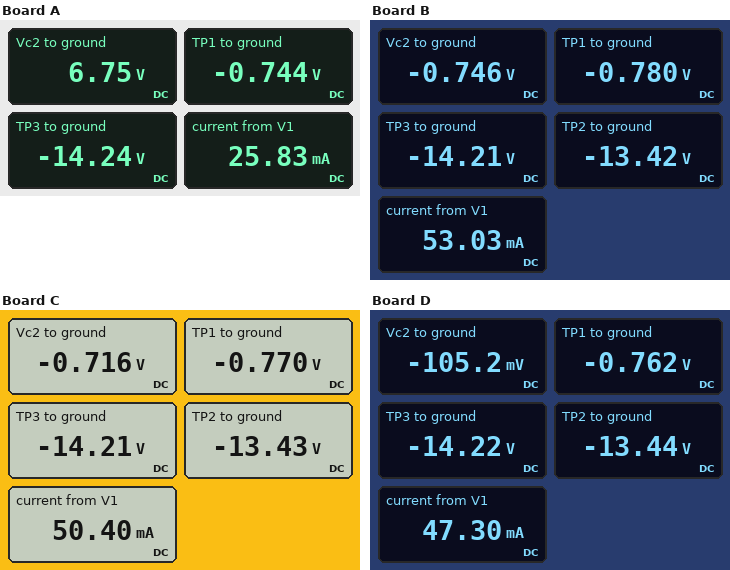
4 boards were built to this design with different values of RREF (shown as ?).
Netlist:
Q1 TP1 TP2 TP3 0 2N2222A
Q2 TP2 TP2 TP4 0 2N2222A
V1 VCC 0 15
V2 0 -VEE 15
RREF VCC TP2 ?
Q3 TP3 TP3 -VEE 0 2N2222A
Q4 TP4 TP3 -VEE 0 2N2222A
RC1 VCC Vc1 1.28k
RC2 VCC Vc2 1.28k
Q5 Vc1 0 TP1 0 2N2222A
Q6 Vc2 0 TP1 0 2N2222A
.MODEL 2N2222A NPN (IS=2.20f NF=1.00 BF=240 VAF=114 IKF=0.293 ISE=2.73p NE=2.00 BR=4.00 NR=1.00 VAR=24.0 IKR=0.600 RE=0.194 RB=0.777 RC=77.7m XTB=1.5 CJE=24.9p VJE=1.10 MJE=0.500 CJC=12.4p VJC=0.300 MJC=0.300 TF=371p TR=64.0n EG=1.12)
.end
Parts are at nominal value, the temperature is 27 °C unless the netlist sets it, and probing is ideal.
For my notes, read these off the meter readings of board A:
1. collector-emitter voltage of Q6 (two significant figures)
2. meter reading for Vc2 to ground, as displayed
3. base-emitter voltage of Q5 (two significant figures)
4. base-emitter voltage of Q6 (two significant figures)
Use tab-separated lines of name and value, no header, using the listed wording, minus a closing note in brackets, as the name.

collector-emitter voltage of Q6	7.5 V
meter reading for Vc2 to ground, as displayed	6.75 V
base-emitter voltage of Q5	740 mV
base-emitter voltage of Q6	740 mV
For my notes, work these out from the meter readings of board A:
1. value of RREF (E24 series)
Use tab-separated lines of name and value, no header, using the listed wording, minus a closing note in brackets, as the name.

value of RREF	2.2 kΩ
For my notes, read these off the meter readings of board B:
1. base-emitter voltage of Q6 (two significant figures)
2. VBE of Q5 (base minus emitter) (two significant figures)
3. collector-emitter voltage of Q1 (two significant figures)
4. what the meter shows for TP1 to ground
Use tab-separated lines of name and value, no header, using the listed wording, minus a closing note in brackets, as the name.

base-emitter voltage of Q6	780 mV
VBE of Q5 (base minus emitter)	780 mV
collector-emitter voltage of Q1	13 V
what the meter shows for TP1 to ground	-0.780 V
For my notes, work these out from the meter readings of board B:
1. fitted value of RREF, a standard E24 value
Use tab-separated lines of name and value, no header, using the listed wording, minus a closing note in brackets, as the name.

fitted value of RREF, a standard E24 value	1 kΩ
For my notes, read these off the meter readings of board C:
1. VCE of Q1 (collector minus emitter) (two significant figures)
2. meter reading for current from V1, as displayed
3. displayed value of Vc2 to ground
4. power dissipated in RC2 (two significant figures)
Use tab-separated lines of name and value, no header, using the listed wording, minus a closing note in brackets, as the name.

VCE of Q1 (collector minus emitter)	13 V
meter reading for current from V1, as displayed	50.40 mA
displayed value of Vc2 to ground	-0.716 V
power dissipated in RC2	190 mW
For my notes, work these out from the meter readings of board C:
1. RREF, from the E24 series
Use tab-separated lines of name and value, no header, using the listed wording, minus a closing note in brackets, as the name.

RREF, from the E24 series	1.1 kΩ
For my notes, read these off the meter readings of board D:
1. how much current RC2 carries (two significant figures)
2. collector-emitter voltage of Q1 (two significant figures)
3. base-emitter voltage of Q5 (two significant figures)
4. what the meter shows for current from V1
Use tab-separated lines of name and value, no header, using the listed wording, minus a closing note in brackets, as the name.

how much current RC2 carries	12 mA
collector-emitter voltage of Q1	13 V
base-emitter voltage of Q5	760 mV
what the meter shows for current from V1	47.30 mA
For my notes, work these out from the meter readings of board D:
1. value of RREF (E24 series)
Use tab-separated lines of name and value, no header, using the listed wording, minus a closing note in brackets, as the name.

value of RREF	1.2 kΩ
